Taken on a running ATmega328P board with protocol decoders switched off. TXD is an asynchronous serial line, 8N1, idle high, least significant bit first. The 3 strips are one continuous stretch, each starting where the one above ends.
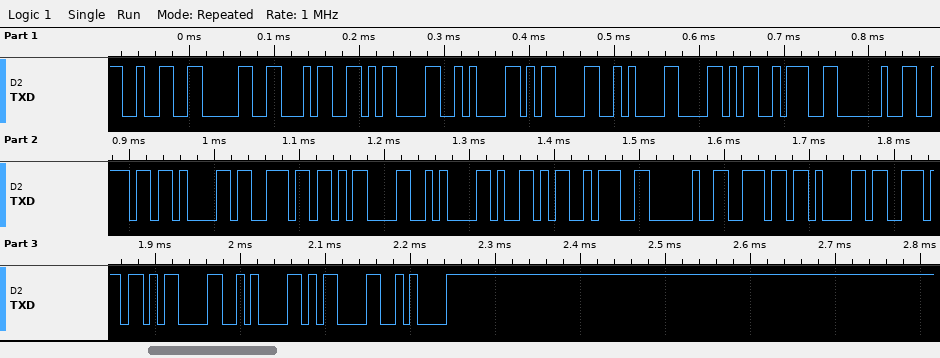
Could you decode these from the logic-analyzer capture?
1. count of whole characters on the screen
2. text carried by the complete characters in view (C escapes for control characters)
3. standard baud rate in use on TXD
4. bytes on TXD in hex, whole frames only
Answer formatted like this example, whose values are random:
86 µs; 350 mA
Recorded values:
25; "204\r\n\r\nX: nan\r\nY: nan\r\n\r\n"; 115200 baud; 0x32 0x30 0x34 0x0D 0x0A 0x0D 0x0A 0x58 0x3A 0x20 0x6E 0x61 0x6E 0x0D 0x0A 0x59 0x3A 0x20 0x6E 0x61 0x6E 0x0D 0x0A 0x0D 0x0A
